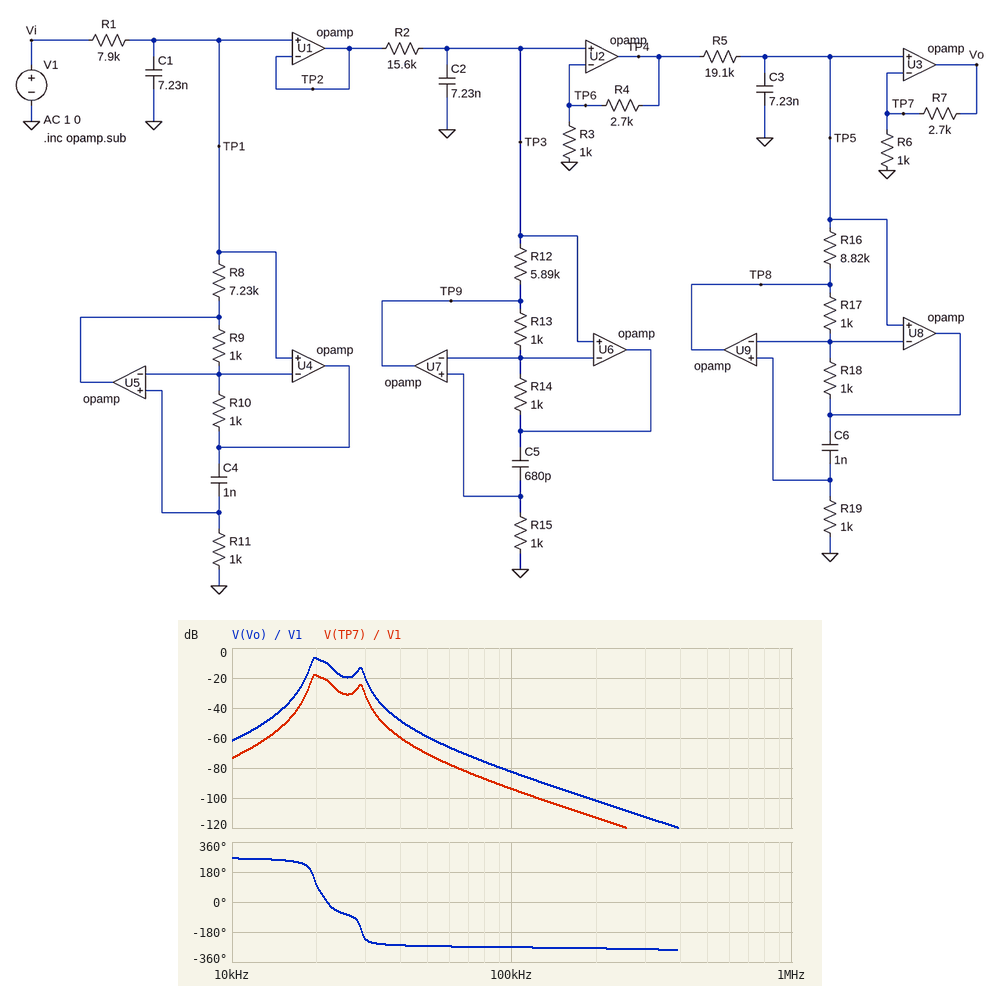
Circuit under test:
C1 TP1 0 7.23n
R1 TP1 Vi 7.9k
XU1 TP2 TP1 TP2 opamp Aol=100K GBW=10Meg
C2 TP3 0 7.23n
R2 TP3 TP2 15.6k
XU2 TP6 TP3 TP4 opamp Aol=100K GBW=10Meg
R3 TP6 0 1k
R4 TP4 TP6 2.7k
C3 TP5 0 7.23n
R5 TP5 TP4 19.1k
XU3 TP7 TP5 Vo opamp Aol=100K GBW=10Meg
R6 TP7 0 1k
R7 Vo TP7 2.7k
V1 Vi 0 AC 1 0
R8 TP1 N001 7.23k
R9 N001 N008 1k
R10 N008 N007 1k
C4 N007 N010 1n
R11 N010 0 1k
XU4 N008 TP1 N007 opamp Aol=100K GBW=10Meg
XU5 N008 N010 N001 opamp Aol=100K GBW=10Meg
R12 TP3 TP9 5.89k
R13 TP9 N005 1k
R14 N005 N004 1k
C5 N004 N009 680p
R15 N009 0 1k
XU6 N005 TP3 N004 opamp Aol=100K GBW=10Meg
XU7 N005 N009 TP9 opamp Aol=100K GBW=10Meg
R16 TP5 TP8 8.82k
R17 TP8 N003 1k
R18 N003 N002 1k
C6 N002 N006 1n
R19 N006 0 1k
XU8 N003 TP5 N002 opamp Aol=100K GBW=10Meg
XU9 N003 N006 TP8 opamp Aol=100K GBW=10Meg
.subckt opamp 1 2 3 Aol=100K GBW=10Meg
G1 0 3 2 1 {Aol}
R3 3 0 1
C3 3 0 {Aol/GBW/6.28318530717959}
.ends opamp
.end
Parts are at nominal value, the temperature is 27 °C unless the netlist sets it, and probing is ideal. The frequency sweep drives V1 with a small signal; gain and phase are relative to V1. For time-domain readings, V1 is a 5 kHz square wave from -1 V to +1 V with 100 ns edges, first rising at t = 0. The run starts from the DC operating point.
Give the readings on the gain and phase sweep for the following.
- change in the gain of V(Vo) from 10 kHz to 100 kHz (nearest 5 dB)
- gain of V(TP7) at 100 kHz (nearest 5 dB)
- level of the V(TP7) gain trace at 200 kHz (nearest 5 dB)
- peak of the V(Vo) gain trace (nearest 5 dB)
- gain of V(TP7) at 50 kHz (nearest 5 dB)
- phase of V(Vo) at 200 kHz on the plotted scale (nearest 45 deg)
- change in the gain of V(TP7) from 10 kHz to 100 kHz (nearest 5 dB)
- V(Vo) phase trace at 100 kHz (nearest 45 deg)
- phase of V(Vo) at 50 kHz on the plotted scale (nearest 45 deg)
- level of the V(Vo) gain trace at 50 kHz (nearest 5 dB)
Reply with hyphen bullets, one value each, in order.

- -20 dB
- -95 dB
- -115 dB
- -5 dB
- -70 dB
- -270 deg
- -20 dB
- -270 deg
- -270 deg
- -60 dB
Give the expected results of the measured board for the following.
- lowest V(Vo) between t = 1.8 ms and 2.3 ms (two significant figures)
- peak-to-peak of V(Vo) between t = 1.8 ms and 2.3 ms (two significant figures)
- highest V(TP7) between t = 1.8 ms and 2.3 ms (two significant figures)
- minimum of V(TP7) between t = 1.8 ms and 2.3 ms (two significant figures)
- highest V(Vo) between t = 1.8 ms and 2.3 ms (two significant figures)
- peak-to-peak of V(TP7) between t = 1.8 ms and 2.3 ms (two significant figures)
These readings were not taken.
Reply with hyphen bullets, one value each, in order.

- -31 mV
- 62 mV
- 8.4 mV
- -8.4 mV
- 31 mV
- 17 mV
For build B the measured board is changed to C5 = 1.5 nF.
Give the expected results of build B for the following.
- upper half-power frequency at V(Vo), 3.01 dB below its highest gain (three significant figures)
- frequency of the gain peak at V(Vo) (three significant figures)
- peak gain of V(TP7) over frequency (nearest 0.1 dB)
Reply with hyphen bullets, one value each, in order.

- 20.2 kHz
- 19.7 kHz
- 6.2 dB
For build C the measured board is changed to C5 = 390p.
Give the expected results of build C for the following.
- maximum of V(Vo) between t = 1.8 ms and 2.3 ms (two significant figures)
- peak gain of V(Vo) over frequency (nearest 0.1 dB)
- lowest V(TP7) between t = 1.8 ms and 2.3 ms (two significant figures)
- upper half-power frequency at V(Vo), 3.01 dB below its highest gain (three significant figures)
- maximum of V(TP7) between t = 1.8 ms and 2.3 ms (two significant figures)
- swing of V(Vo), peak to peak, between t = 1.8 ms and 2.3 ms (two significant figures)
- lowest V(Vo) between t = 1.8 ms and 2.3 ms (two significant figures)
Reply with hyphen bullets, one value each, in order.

- 12 mV
- -13.7 dB
- -3.3 mV
- 21.1 kHz
- 3.3 mV
- 24 mV
- -12 mV
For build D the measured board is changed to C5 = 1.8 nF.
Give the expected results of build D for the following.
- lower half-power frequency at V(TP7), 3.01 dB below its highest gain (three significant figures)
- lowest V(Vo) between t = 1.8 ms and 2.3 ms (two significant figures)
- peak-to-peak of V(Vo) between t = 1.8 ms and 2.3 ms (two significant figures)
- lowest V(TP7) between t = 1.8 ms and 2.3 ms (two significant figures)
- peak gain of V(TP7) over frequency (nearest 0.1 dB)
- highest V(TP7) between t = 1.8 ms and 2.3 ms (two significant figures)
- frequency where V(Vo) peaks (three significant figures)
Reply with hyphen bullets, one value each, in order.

- 18.8 kHz
- -41 mV
- 81 mV
- -11 mV
- -1.6 dB
- 11 mV
- 19.6 kHz
